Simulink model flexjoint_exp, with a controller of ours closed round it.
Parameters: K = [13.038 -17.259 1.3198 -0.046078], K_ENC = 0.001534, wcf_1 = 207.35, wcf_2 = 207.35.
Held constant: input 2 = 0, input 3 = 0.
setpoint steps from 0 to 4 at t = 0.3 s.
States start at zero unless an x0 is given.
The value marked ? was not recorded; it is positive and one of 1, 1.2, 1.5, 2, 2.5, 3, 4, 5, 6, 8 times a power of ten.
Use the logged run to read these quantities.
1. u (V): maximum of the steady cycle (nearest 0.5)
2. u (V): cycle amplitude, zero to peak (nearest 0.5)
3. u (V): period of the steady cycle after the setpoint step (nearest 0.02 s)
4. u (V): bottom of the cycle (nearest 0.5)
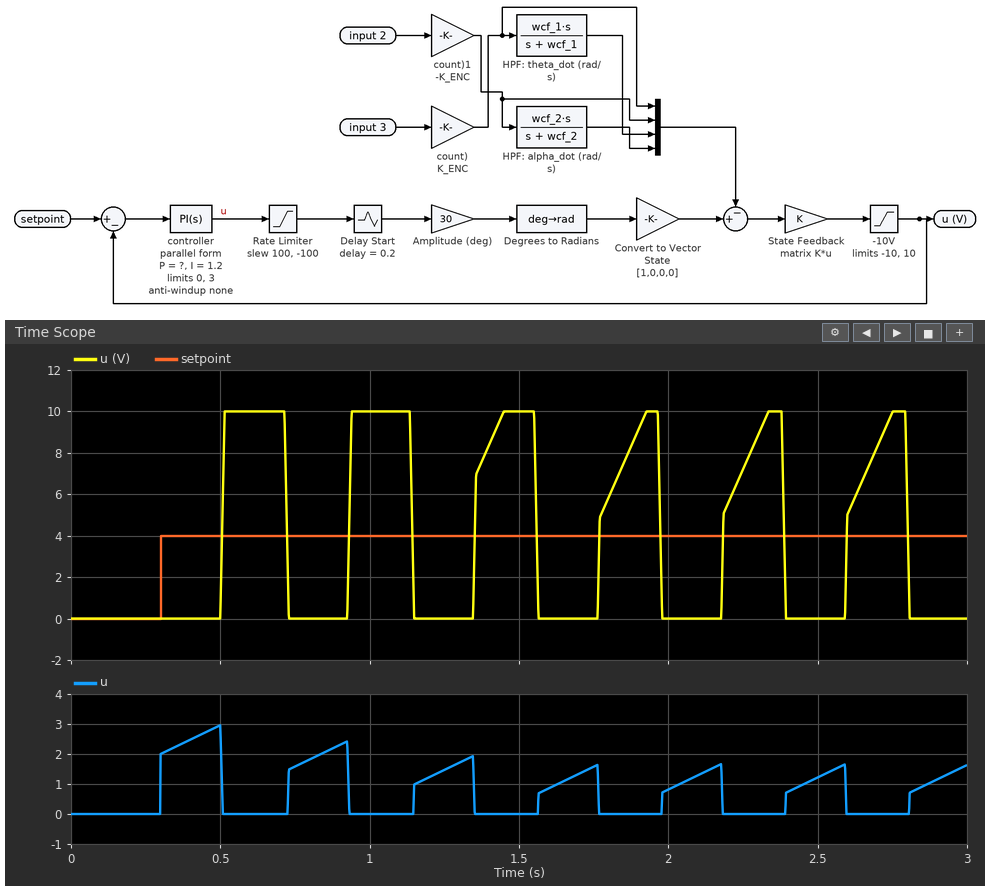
10.0
5.0
0.42 s
0.0
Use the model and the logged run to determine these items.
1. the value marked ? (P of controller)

0.5
